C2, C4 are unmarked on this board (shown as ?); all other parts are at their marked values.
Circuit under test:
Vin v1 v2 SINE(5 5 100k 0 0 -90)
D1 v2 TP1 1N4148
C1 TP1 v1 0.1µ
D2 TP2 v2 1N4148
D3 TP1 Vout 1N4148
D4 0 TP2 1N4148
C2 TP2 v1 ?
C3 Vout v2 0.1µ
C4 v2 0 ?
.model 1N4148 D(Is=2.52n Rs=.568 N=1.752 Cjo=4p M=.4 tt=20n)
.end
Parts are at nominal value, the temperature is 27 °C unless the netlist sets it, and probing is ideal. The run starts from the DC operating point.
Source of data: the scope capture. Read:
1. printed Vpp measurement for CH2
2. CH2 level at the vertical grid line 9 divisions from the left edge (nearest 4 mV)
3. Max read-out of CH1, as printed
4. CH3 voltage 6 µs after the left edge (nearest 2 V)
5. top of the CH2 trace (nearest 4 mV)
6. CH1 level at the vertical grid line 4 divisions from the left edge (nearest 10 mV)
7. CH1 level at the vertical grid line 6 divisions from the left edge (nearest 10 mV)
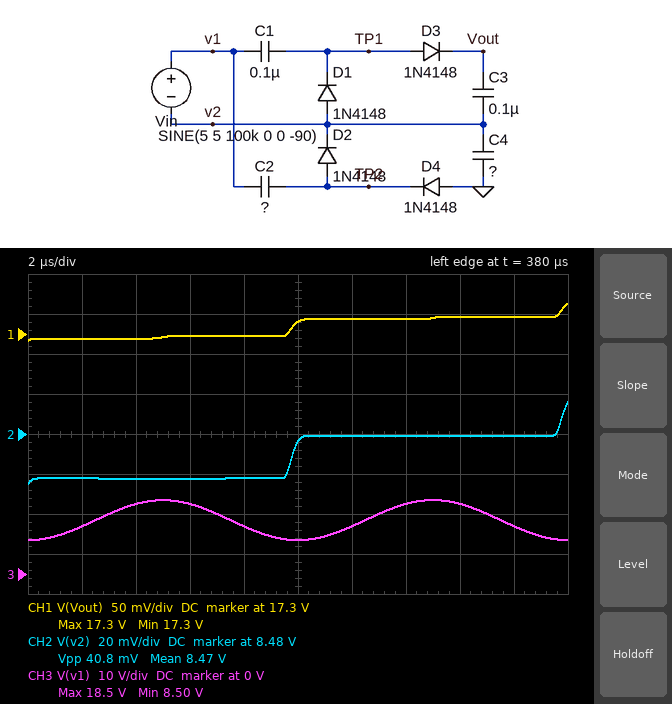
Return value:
40.8 mV
8.480 V
17.3 V
18 V
8.496 V
17.30 V
17.32 V
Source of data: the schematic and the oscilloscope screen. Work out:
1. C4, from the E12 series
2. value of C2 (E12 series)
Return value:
330 nF
33 nF
